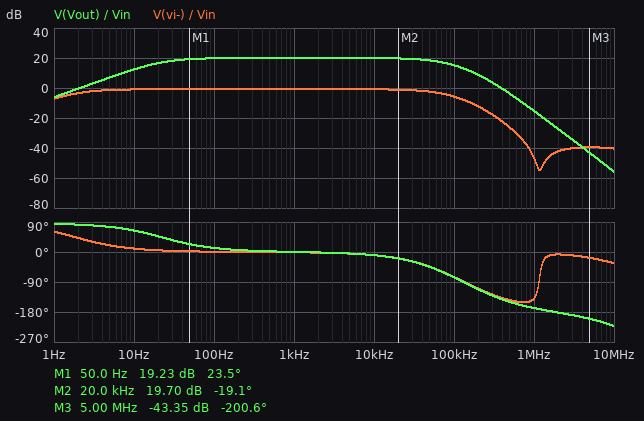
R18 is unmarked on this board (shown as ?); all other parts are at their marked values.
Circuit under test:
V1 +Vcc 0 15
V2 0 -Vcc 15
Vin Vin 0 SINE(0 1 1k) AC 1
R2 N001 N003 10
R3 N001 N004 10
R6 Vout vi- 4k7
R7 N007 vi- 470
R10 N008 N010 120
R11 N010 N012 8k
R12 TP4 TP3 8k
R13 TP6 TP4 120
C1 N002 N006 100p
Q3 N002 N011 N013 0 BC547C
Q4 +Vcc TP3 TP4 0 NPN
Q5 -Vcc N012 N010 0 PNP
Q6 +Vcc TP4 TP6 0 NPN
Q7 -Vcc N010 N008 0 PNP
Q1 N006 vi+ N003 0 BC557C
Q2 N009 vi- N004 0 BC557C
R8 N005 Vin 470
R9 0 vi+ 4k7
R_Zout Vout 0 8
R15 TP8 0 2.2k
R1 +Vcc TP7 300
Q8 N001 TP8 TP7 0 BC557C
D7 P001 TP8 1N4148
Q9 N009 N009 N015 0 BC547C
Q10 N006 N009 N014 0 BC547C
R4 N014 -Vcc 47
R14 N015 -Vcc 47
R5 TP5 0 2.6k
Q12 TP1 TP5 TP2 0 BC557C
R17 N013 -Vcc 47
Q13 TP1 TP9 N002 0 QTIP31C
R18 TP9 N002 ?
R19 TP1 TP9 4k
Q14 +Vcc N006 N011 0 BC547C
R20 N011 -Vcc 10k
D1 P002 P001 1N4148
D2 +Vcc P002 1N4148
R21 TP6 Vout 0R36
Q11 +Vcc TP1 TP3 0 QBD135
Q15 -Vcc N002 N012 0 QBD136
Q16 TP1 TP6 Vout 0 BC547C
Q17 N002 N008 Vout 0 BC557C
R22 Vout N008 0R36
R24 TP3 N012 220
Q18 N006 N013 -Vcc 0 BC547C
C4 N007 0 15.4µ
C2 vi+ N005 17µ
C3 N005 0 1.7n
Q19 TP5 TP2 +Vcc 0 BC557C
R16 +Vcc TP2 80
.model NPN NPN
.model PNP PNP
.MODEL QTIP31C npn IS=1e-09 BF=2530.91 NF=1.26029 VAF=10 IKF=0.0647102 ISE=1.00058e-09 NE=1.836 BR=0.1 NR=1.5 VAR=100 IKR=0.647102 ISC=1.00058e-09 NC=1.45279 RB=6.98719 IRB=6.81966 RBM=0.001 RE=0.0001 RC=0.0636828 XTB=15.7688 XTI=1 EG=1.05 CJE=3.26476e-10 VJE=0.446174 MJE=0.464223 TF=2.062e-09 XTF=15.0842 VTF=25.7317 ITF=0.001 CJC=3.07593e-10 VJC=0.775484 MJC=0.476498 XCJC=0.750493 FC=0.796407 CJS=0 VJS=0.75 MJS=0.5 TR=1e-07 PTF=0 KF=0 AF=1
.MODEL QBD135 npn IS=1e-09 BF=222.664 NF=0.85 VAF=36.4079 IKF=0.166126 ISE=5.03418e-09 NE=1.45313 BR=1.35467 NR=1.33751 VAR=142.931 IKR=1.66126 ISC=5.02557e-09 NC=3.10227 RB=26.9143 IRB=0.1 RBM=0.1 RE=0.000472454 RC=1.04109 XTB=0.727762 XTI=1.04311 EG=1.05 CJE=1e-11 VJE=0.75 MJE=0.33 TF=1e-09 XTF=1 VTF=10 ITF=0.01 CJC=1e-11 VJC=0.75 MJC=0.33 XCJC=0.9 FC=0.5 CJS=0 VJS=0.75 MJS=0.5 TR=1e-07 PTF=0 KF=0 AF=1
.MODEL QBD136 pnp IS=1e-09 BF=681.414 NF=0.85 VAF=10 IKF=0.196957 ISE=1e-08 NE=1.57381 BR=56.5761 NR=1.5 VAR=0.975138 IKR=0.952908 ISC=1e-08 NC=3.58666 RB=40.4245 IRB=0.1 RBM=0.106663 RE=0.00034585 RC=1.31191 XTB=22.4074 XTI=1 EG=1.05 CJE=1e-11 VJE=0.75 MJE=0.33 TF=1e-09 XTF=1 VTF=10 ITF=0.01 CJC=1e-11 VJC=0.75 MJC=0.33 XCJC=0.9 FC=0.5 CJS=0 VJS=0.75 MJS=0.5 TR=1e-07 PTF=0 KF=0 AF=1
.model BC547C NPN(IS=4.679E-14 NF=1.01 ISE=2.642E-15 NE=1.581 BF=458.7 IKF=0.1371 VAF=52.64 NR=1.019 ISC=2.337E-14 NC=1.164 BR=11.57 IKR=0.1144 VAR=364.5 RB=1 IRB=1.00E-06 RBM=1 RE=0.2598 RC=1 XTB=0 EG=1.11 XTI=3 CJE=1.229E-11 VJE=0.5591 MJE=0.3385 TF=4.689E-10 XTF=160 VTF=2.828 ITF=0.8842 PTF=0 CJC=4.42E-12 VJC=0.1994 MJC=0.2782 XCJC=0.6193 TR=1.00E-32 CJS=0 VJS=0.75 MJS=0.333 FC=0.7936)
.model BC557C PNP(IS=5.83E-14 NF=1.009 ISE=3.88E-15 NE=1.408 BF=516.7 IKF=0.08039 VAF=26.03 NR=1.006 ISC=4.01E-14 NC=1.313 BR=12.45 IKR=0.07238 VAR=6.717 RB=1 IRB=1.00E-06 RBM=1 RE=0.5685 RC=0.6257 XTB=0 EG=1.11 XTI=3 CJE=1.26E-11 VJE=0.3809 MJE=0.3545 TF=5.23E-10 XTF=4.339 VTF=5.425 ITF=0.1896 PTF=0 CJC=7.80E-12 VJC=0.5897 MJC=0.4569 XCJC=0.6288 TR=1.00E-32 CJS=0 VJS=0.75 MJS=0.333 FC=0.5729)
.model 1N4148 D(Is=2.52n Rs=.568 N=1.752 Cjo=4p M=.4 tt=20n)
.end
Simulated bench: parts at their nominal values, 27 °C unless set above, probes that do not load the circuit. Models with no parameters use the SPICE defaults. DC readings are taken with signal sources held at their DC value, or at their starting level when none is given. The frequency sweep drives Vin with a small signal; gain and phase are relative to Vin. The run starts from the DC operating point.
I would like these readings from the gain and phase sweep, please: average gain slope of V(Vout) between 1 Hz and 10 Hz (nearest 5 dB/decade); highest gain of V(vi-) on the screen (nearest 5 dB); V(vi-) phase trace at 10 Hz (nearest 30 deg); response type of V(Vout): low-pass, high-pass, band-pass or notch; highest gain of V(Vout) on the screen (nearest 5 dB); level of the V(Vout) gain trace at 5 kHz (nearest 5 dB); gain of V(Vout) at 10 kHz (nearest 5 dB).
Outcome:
20 dB/decade
0 dB
0 deg
band-pass
20 dB
20 dB
20 dB
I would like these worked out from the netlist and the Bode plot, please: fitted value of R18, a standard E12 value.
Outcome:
2.7 kΩ
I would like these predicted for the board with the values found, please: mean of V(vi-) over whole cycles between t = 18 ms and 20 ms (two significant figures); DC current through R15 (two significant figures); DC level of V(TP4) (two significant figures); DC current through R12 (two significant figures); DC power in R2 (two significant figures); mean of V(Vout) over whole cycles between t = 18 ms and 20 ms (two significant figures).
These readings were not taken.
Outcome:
-200 mV
5.9 mA
17 mV
87 µA
51 µW
-640 mV
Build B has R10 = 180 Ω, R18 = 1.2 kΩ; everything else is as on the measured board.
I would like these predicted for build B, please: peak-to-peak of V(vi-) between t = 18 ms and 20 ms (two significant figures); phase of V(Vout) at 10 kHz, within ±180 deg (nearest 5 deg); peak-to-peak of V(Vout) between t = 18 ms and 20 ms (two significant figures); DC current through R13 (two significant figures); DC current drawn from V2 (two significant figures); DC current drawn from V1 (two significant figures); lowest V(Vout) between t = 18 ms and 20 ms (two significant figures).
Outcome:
1.8 V
-5 deg
20 V
850 µA
22 mA
33 mA
-10 V
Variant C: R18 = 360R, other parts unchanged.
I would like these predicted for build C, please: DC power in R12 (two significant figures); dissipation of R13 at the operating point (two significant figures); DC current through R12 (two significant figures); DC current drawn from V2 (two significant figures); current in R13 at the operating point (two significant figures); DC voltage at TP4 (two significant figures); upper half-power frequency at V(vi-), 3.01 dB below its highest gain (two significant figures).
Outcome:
92 µW
7.8 mW
110 µA
1.9 A
8.1 mA
1.6 V
220 kHz
